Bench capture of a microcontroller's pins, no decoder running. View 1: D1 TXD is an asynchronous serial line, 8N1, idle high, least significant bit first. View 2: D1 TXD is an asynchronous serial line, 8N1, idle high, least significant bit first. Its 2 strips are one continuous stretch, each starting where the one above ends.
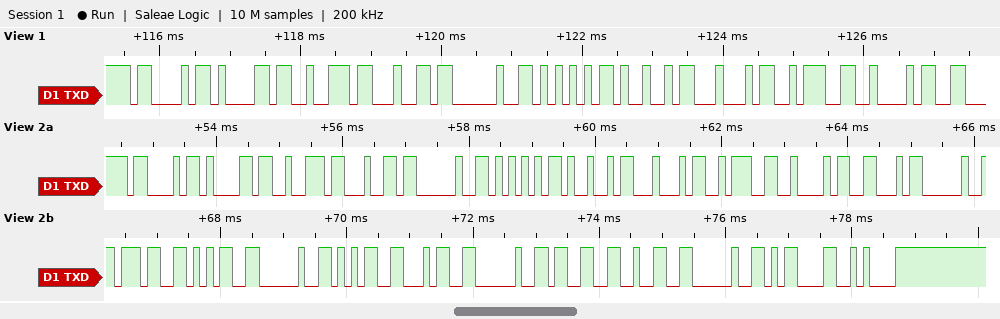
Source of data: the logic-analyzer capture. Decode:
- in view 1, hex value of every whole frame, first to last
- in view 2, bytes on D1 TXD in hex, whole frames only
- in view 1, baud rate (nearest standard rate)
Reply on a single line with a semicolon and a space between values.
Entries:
43 61 72 64 20 55 49 44 3A 42; 43 61 72 64 20 55 49 44 3A 42 46 20 37 35 20 35 34 20 33 32 20 0D 0A; 9600 baud
